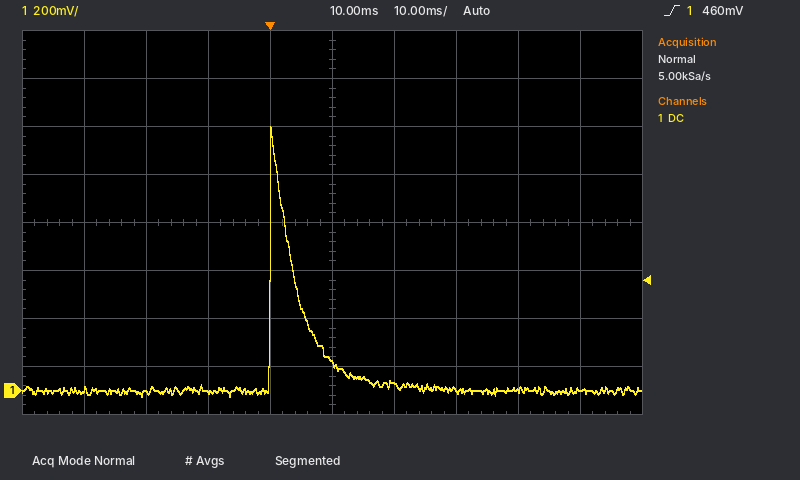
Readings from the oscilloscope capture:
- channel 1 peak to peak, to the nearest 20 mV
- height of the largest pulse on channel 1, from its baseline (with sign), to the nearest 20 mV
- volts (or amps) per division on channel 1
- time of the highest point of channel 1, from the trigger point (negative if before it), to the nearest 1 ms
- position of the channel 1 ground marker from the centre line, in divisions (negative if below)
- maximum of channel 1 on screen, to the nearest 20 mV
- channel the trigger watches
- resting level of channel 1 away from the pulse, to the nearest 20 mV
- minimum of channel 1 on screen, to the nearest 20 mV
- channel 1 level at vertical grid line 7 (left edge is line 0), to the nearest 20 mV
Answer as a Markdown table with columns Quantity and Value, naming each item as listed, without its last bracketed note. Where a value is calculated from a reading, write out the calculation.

| Quantity | Value |
|---|---|
| channel 1 peak to peak, to the nearest 20 mV | 1.10 V − (-20 mV) = 1.12 V |
| height of the largest pulse on channel 1, from its baseline (with sign), to the nearest 20 mV | 1.10 V − (0 mV) = +1.10 V |
| volts (or amps) per division on channel 1 | 200 mV |
| time of the highest point of channel 1, from the trigger point (negative if before it), to the nearest 1 ms | 0 ms |
| position of the channel 1 ground marker from the centre line, in divisions | -3.5 div |
| maximum of channel 1 on screen, to the nearest 20 mV | 1.10 V |
| channel the trigger watches | channel 1 |
| resting level of channel 1 away from the pulse, to the nearest 20 mV | 0 mV |
| minimum of channel 1 on screen, to the nearest 20 mV | -20 mV |
| channel 1 level at vertical grid line 7 (left edge is line 0), to the nearest 20 mV | 0 mV |
